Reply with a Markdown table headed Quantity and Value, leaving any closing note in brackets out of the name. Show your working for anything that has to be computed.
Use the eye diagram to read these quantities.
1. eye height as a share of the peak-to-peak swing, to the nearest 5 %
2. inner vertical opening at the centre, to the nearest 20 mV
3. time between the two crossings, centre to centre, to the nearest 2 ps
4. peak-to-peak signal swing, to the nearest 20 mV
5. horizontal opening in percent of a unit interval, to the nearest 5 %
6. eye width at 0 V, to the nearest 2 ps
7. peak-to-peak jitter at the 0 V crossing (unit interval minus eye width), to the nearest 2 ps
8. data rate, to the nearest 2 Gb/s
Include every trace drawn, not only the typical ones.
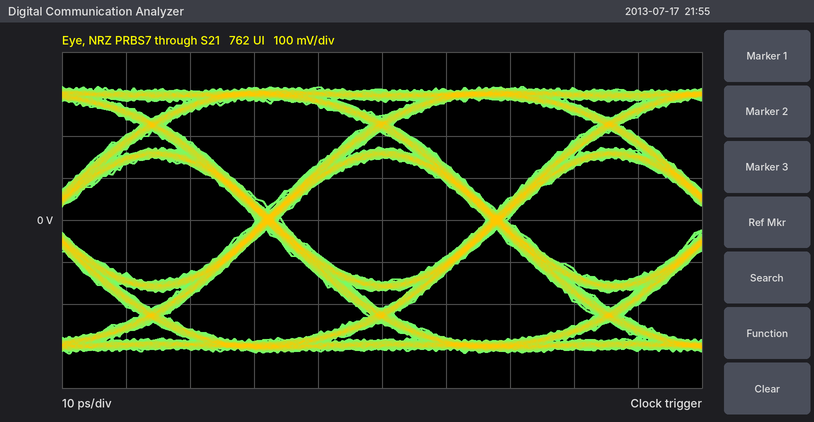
| Quantity | Value |
|---|---|
| eye height as a share of the peak-to-peak swing, to the nearest 5 % | 300 mV / 640 mV ≈ 46.9 %, so 45 % to the nearest 5 % |
| inner vertical opening at the centre, to the nearest 20 mV | 300 mV |
| time between the two crossings, centre to centre, to the nearest 2 ps | 36 ps |
| peak-to-peak signal swing, to the nearest 20 mV | 640 mV |
| horizontal opening in percent of a unit interval, to the nearest 5 % | 32 ps / 36 ps ≈ 88.9 %, so 90 % to the nearest 5 % |
| eye width at 0 V, to the nearest 2 ps | 32 ps |
| peak-to-peak jitter at the 0 V crossing (unit interval minus eye width), to the nearest 2 ps | 4 ps |
| data rate, to the nearest 2 Gb/s | 28 Gb/s |
